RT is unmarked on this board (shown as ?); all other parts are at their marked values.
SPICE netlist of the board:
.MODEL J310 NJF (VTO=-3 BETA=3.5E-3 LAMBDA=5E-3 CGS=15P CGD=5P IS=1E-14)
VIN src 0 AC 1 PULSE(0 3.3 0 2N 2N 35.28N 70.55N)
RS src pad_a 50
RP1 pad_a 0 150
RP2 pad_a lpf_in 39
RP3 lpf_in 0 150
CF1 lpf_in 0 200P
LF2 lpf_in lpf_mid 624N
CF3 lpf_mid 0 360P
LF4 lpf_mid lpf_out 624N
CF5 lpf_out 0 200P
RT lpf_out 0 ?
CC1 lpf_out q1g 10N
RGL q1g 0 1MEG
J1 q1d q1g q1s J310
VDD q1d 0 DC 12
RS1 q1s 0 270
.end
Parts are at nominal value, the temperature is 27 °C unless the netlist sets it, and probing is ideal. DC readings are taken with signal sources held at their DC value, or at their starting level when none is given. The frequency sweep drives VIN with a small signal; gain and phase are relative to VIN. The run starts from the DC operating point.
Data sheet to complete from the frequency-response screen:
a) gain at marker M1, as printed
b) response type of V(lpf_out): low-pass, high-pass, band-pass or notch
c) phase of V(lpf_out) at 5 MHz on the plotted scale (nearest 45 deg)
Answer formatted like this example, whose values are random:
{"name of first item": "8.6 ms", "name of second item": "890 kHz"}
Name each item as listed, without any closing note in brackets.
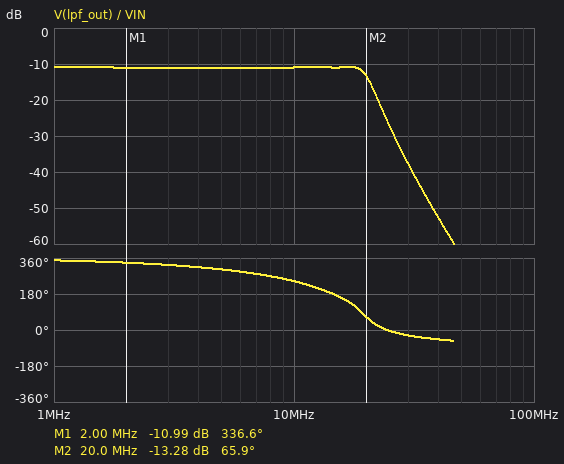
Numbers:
{"gain at marker M1, as printed": "-10.99 dB", "response type of V(lpf_out): low-pass, high-pass, band-pass or notch": "low-pass", "phase of V(lpf_out) at 5 MHz on the plotted scale": "315 deg"}
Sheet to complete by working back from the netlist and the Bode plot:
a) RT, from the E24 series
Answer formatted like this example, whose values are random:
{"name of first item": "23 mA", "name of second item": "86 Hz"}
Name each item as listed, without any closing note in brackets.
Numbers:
{"RT, from the E24 series": "68 Ω"}
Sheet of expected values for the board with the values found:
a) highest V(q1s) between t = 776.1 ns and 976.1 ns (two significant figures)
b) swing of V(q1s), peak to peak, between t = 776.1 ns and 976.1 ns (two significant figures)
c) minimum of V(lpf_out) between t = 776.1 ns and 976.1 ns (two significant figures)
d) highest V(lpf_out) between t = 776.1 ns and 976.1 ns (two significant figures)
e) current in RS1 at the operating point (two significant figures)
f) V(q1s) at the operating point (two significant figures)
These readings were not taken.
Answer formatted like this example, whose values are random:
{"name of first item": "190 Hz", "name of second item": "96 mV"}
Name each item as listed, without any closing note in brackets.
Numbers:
{"highest V(q1s) between t = 776.1 ns and 976.1 ns": "2.5 V", "swing of V(q1s), peak to peak, between t = 776.1 ns and 976.1 ns": "870 mV", "minimum of V(lpf_out) between t = 776.1 ns and 976.1 ns": "-98 mV", "highest V(lpf_out) between t = 776.1 ns and 976.1 ns": "1.1 V", "current in RS1 at the operating point": "6.3 mA", "V(q1s) at the operating point": "1.7 V"}
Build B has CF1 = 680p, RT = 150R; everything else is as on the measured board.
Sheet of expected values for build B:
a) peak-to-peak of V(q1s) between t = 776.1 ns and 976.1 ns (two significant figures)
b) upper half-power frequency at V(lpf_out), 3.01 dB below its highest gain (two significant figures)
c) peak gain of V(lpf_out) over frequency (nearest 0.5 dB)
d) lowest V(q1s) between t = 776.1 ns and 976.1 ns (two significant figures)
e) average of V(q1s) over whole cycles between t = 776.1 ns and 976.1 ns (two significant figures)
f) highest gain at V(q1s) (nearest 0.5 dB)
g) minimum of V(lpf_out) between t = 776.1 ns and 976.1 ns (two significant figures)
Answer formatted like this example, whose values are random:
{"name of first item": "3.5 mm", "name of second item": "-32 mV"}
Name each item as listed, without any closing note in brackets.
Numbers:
{"peak-to-peak of V(q1s) between t = 776.1 ns and 976.1 ns": "600 mV", "upper half-power frequency at V(lpf_out), 3.01 dB below its highest gain": "12 MHz", "peak gain of V(lpf_out) over frequency": "-7.5 dB", "lowest V(q1s) between t = 776.1 ns and 976.1 ns": "1.9 V", "average of V(q1s) over whole cycles between t = 776.1 ns and 976.1 ns": "2.2 V", "highest gain at V(q1s)": "-10.5 dB", "minimum of V(lpf_out) between t = 776.1 ns and 976.1 ns": "240 mV"}
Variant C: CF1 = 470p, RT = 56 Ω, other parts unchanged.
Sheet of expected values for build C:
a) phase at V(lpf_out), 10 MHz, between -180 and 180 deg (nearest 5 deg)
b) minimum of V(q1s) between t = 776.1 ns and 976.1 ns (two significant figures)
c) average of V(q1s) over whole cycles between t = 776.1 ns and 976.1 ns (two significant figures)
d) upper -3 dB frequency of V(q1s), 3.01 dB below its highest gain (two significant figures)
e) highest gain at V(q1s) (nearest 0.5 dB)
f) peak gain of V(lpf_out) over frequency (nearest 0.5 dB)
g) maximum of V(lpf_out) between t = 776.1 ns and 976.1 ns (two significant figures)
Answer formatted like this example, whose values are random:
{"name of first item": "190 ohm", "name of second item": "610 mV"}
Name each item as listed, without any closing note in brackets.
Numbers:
{"phase at V(lpf_out), 10 MHz, between -180 and 180 deg": "-140 deg", "minimum of V(q1s) between t = 776.1 ns and 976.1 ns": "1.7 V", "average of V(q1s) over whole cycles between t = 776.1 ns and 976.1 ns": "2.0 V", "upper -3 dB frequency of V(q1s), 3.01 dB below its highest gain": "18 MHz", "highest gain at V(q1s)": "-14.5 dB", "peak gain of V(lpf_out) over frequency": "-11.5 dB", "maximum of V(lpf_out) between t = 776.1 ns and 976.1 ns": "890 mV"}
